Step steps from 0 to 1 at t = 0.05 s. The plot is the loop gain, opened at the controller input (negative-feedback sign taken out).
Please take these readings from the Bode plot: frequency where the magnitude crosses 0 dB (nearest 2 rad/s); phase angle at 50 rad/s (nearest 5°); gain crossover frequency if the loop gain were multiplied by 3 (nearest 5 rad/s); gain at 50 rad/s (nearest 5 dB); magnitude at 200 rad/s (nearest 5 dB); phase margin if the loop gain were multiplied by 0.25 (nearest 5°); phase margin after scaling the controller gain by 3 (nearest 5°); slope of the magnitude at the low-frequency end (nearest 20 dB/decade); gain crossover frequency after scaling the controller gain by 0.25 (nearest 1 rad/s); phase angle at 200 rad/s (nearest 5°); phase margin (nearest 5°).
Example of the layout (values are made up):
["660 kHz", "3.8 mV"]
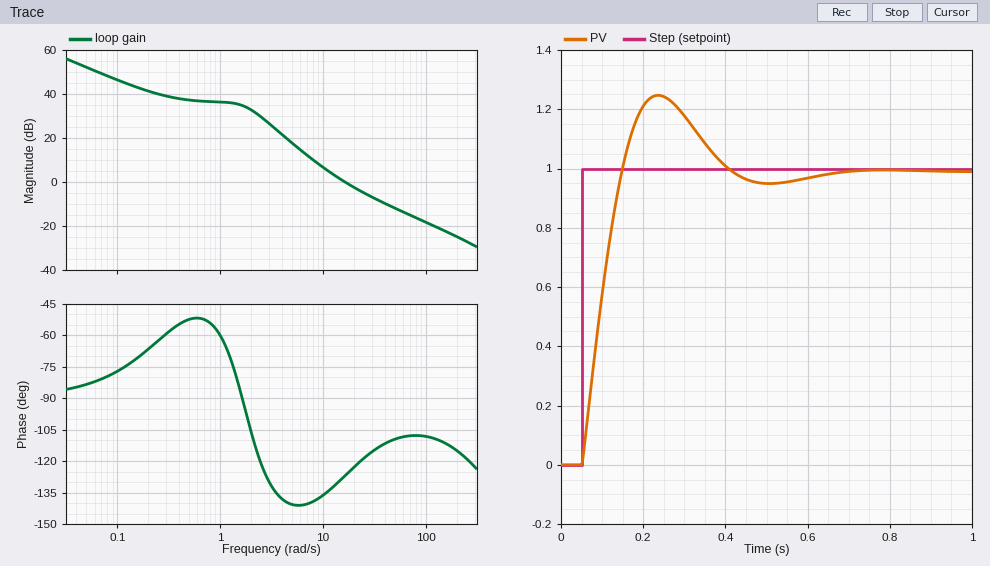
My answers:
["16 rad/s", "-110°", "40 rad/s", "-10 dB", "-25 dB", "40°", "70°", "-20 dB/decade", "7 rad/s", "-115°", "55°"]
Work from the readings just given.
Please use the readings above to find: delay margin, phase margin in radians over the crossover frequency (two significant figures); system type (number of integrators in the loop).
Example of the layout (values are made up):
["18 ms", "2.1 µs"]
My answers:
["0.060 s", "1"]
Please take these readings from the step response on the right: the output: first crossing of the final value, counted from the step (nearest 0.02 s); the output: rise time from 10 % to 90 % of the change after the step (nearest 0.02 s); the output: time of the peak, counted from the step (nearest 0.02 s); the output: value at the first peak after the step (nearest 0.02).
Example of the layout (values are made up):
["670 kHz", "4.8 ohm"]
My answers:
["0.10 s", "0.08 s", "0.18 s", "1.24"]
